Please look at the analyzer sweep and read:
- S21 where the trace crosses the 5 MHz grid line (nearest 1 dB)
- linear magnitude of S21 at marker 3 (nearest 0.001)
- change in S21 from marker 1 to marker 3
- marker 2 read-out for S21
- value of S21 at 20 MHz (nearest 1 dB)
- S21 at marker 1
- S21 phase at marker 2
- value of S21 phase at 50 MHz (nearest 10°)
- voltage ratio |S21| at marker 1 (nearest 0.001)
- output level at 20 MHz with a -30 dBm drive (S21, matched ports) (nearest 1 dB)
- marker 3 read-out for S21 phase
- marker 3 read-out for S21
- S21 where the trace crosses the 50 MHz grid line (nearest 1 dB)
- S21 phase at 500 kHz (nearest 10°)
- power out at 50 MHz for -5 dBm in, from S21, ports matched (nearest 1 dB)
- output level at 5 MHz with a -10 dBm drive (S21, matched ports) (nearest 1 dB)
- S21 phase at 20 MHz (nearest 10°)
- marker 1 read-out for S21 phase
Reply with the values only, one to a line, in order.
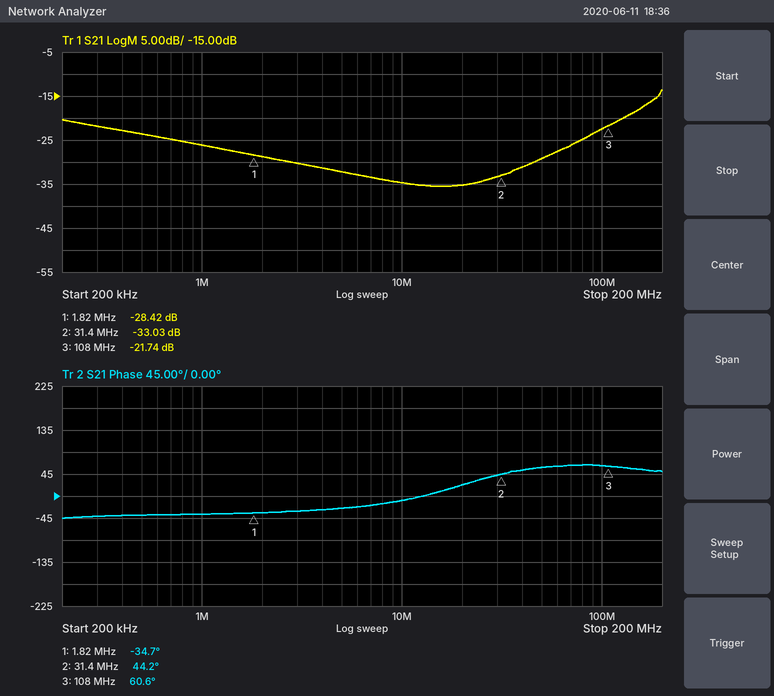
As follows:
-32 dB
0.082
6.68 dB
-33.03 dB
-35 dB
-28.42 dB
44.2°
60°
0.038
-65 dBm
60.6°
-21.74 dB
-29 dB
-40°
-34 dBm
-42 dBm
20°
-34.7°
